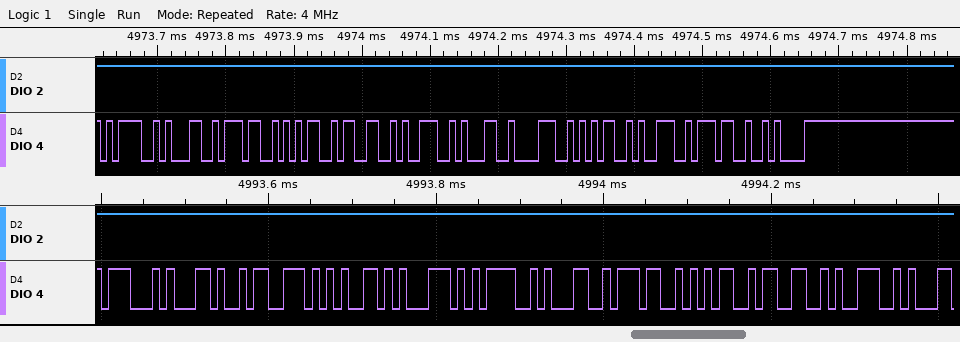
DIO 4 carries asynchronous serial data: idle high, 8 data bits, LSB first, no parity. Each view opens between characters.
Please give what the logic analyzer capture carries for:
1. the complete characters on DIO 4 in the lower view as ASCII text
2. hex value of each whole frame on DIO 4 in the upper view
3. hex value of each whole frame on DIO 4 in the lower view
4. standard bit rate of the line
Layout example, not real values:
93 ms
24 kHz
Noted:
"G,seq=17539"
3D, 31, 37, 35, 33, 39, 31, 38, 35, 39, 37, 0A
47, 2C, 73, 65, 71, 3D, 31, 37, 35, 33, 39
115200 baud
